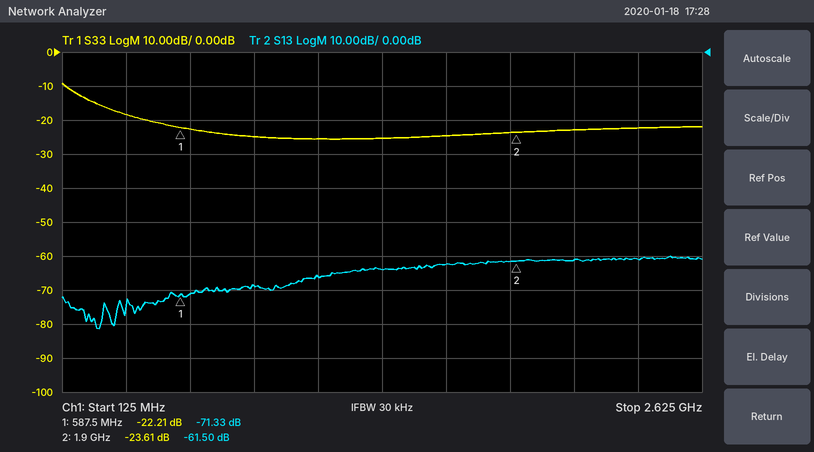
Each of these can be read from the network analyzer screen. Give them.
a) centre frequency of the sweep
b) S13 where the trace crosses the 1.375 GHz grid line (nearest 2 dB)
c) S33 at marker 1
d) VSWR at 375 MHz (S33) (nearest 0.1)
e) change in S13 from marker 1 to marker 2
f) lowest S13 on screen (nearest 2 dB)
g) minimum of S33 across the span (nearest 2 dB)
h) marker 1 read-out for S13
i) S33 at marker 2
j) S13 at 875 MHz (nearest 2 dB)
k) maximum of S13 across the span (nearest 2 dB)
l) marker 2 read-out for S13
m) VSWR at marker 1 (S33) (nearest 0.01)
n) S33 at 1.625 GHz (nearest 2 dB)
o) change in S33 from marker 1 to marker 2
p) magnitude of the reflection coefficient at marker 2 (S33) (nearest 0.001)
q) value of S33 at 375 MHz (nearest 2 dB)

1.375 GHz
-64 dB
-22.21 dB
1.3
9.83 dB
-82 dB
-26 dB
-71.33 dB
-23.61 dB
-68 dB
-60 dB
-61.50 dB
1.17
-24 dB
-1.40 dB
0.066
-18 dB
